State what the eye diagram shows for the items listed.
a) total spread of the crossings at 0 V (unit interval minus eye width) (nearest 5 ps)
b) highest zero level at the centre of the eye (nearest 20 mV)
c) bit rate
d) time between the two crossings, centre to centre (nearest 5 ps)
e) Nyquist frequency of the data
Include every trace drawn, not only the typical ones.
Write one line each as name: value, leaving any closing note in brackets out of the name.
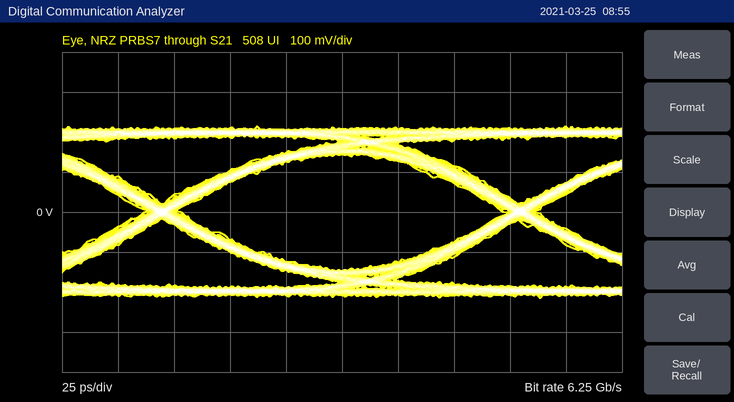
total spread of the crossings at 0 V (unit interval minus eye width): 15 ps
highest zero level at the centre of the eye: -140 mV
bit rate: 6.25 Gb/s
time between the two crossings, centre to centre: 160 ps
Nyquist frequency of the data: 3.125 GHz
